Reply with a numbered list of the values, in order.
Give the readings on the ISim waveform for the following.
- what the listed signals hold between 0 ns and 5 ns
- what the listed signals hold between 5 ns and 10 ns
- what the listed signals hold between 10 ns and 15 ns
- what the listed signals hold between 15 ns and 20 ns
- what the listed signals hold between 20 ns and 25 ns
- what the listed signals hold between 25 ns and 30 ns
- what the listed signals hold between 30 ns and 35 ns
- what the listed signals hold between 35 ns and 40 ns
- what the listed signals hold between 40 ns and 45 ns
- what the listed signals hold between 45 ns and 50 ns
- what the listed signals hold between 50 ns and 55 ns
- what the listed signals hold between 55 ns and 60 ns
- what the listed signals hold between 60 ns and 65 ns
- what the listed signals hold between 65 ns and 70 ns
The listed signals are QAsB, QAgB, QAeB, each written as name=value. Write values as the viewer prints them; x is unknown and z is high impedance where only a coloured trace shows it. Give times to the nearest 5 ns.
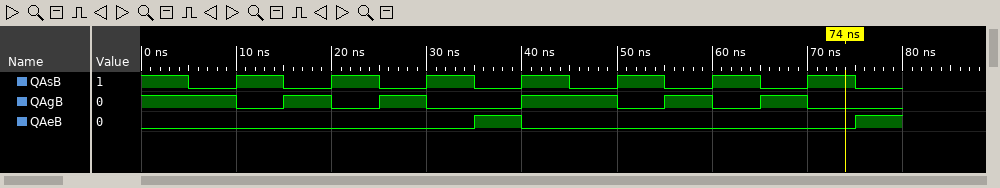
1. QAsB=1, QAgB=1, QAeB=0
2. QAsB=0, QAgB=1, QAeB=0
3. QAsB=1, QAgB=0, QAeB=0
4. QAsB=0, QAgB=1, QAeB=0
5. QAsB=1, QAgB=0, QAeB=0
6. QAsB=0, QAgB=1, QAeB=0
7. QAsB=1, QAgB=0, QAeB=0
8. QAsB=0, QAgB=0, QAeB=1
9. QAsB=1, QAgB=1, QAeB=0
10. QAsB=0, QAgB=1, QAeB=0
11. QAsB=1, QAgB=0, QAeB=0
12. QAsB=0, QAgB=1, QAeB=0
13. QAsB=1, QAgB=0, QAeB=0
14. QAsB=0, QAgB=1, QAeB=0
